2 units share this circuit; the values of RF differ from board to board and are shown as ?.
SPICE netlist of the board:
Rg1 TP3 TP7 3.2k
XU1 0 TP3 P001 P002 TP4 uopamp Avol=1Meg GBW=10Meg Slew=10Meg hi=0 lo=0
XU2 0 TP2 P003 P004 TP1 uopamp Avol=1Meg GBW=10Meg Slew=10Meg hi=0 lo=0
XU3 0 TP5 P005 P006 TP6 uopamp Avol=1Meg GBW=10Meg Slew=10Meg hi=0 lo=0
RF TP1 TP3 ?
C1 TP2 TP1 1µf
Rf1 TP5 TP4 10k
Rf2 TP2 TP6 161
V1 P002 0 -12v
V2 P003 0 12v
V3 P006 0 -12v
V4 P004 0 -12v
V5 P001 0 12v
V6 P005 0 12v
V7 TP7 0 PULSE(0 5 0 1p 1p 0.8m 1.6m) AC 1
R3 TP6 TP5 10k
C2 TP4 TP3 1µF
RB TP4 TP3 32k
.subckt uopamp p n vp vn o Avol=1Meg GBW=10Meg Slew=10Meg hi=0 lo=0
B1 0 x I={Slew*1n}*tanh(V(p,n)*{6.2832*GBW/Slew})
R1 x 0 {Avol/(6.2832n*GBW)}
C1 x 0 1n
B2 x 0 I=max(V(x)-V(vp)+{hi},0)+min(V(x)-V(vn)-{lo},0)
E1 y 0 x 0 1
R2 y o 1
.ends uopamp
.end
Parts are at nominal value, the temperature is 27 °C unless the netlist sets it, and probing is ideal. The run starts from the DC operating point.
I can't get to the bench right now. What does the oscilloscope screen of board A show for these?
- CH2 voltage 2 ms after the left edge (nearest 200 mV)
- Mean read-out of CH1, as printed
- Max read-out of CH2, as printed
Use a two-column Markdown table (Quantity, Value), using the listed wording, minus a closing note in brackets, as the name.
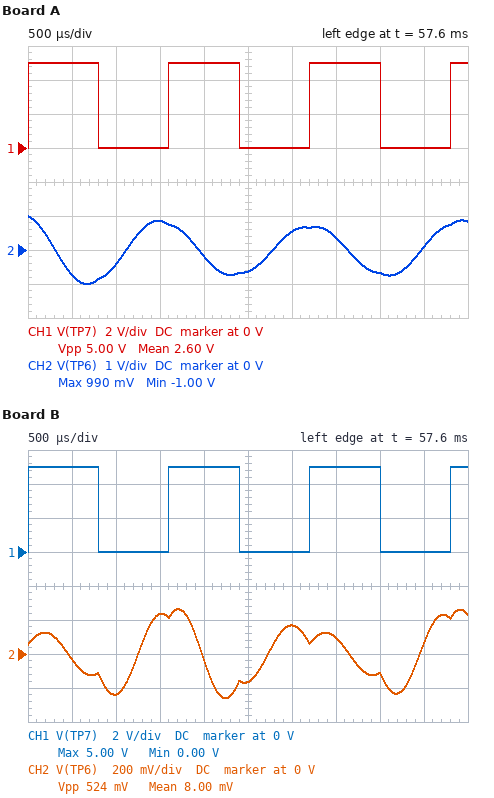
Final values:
| Quantity | Value |
|---|---|
| CH2 voltage 2 ms after the left edge | -200 mV |
| Mean read-out of CH1, as printed | 2.60 V |
| Max read-out of CH2, as printed | 990 mV |
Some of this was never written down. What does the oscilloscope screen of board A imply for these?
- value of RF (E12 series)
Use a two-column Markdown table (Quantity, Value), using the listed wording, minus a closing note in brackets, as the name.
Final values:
| Quantity | Value |
|---|---|
| value of RF | 330 Ω |
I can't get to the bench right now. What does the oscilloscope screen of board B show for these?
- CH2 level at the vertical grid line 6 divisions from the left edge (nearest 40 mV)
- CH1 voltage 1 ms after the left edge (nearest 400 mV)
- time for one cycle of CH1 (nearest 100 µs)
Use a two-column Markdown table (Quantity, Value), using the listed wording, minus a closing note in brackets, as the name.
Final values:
| Quantity | Value |
|---|---|
| CH2 level at the vertical grid line 6 divisions from the left edge | 160 mV |
| CH1 voltage 1 ms after the left edge | 0 V |
| time for one cycle of CH1 | 1.6 ms |
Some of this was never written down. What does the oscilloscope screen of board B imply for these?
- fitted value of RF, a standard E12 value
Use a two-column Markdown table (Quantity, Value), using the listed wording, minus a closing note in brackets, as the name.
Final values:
| Quantity | Value |
|---|---|
| fitted value of RF, a standard E12 value | 180 Ω |
